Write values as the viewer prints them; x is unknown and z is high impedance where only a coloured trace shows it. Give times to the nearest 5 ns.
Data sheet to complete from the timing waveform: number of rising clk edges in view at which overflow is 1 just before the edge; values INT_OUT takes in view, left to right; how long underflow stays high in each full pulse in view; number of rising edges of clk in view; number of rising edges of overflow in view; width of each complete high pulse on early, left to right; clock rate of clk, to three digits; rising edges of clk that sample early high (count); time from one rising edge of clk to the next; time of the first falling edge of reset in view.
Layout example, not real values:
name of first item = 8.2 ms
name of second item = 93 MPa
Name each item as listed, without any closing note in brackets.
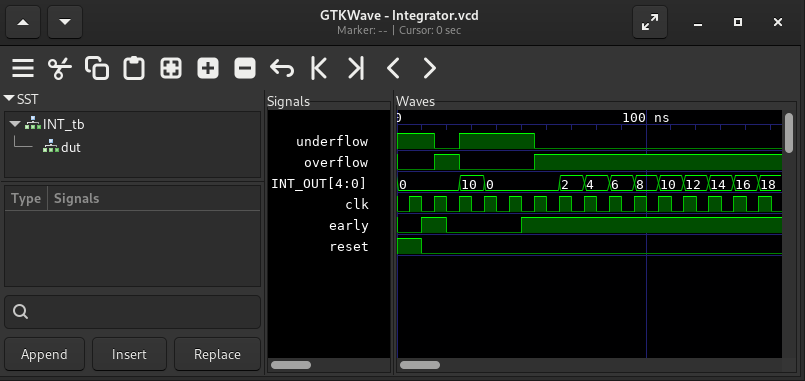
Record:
number of rising clk edges in view at which overflow is 1 just before the edge = 10
values INT_OUT takes in view, left to right = 0, 10, 0, 2, 4, 6, 8, 10, 12, 14, 16, 18
how long underflow stays high in each full pulse in view = 30 ns
number of rising edges of clk in view = 15
number of rising edges of overflow in view = 2
width of each complete high pulse on early, left to right = 10 ns
clock rate of clk, to three digits = 100 MHz
rising edges of clk that sample early high = 11
time from one rising edge of clk to the next = 10 ns
time of the first falling edge of reset in view = 10 ns
